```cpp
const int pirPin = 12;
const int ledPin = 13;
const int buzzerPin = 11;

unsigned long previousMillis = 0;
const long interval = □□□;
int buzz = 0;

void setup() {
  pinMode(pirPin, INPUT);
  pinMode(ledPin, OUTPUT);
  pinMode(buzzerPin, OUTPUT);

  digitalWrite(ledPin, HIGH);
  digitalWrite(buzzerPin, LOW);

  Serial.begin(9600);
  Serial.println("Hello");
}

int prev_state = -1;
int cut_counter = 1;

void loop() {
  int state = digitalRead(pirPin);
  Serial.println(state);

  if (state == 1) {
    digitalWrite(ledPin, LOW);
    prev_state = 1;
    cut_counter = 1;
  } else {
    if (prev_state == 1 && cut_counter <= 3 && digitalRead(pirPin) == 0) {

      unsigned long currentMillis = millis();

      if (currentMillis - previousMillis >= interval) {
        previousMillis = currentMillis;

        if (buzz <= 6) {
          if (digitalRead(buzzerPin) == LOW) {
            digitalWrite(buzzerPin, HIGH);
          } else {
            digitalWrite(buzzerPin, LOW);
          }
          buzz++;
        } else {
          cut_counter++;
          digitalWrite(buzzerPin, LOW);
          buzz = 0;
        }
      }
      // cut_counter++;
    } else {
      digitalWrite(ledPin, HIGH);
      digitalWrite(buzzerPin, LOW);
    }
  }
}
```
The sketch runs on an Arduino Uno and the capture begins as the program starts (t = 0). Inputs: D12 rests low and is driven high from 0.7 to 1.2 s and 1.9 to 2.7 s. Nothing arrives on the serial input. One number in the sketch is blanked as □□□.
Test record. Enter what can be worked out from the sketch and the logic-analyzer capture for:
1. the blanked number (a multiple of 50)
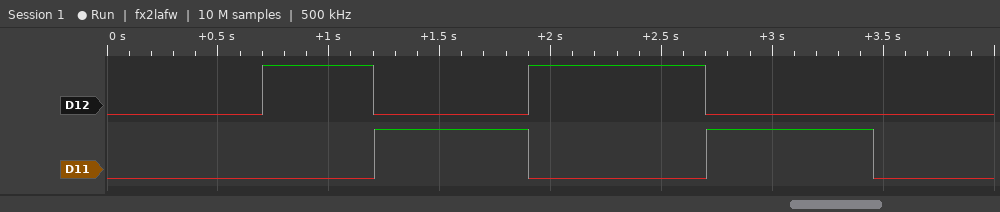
750
